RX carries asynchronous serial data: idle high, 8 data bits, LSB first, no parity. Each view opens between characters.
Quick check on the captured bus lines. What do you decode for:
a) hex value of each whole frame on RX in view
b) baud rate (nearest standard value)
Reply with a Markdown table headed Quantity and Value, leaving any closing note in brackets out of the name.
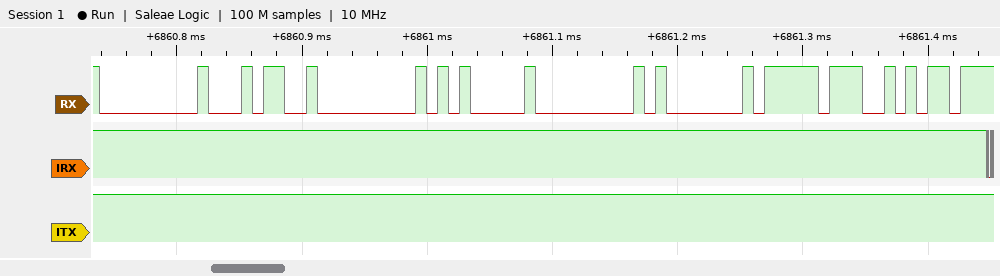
| Quantity | Value |
|---|---|
| hex value of each whole frame on RX in view | 00, 34, 00, 05, 00, 01, DF, 6A |
| baud rate | 115200 baud |
